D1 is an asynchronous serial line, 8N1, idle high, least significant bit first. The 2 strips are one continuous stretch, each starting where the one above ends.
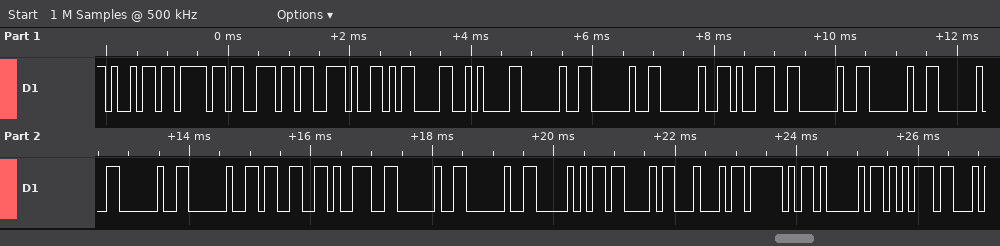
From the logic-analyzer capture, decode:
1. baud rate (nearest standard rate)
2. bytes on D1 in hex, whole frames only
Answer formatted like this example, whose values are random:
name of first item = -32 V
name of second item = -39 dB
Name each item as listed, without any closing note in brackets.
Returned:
baud rate = 9600 baud
bytes on D1 in hex, whole frames only = 69 6F 6E 2E 0D 0A 20 20 20 39 20 20 20 20 20 33 39 20 20 50 43 44 5F 41 75
